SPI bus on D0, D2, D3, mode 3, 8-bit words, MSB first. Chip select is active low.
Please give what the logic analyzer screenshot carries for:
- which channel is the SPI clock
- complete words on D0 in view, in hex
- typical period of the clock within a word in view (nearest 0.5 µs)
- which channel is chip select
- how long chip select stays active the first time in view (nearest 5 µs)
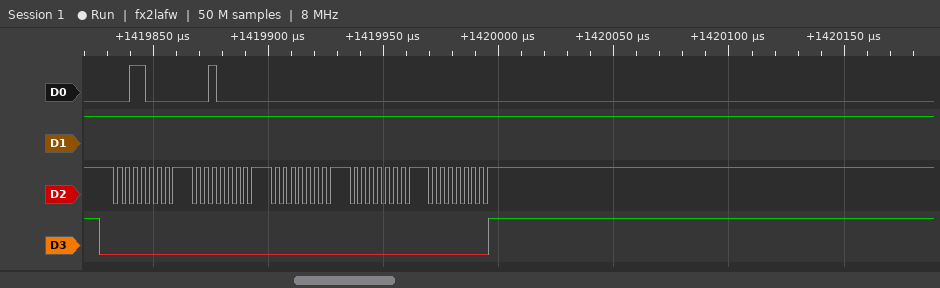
D2
30, 20, 00, 00, 00
3.5 µs
D3
170 µs
